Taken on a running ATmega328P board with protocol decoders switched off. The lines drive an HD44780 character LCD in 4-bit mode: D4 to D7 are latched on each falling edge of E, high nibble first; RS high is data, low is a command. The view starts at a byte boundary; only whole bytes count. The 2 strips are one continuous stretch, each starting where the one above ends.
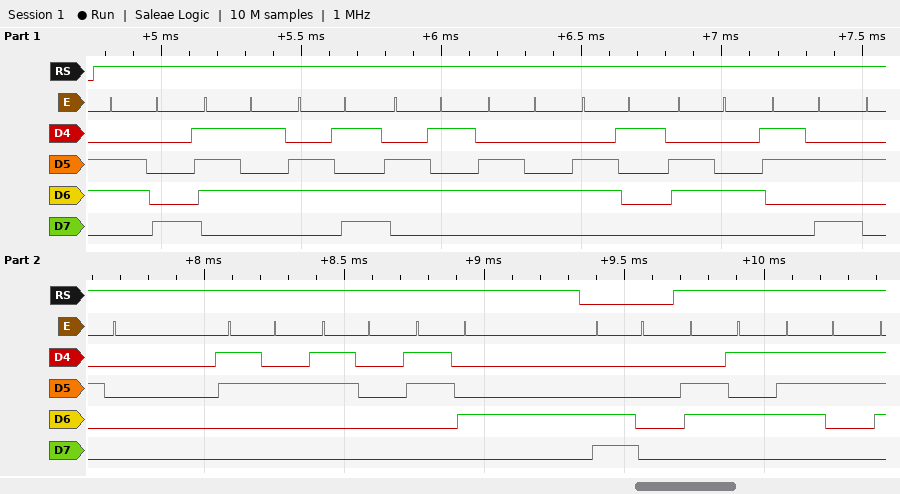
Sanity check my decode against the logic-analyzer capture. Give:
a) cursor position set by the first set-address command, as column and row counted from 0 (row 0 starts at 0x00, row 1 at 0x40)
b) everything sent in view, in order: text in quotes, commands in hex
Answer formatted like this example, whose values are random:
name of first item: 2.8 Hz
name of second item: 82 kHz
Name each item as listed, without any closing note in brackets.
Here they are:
cursor position set by the first set-address command, as column and row counted from 0: column 0, row 1
everything sent in view, in order: text in quotes, commands in hex: "humedad: 204" 0xC0 "es"
